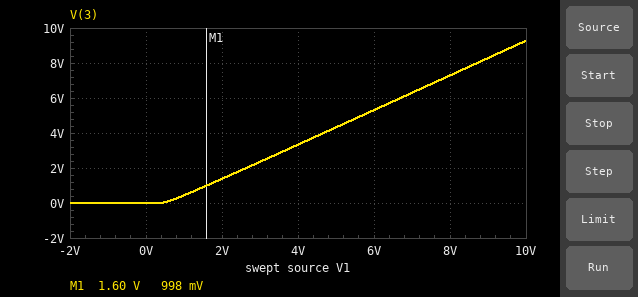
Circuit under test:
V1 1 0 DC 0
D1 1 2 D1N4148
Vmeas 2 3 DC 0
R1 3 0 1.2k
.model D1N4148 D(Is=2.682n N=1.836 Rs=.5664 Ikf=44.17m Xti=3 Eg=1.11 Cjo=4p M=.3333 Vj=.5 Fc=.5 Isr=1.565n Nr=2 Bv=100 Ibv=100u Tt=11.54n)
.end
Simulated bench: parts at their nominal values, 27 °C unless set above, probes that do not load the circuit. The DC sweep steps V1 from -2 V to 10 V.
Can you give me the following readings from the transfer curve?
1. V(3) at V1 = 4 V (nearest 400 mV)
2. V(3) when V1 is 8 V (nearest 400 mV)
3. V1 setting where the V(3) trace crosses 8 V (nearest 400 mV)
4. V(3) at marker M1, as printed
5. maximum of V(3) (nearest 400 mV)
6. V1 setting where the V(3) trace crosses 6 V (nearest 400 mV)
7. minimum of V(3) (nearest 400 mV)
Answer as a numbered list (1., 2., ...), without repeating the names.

1. 3.2 V
2. 7.2 V
3. 8.8 V
4. 998 mV
5. 9.2 V
6. 6.8 V
7. 0 V
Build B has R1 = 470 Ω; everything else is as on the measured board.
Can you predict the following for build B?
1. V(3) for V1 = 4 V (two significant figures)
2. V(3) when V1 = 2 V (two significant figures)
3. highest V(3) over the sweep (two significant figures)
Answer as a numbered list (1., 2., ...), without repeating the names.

1. 3.3 V
2. 1.3 V
3. 9.2 V
